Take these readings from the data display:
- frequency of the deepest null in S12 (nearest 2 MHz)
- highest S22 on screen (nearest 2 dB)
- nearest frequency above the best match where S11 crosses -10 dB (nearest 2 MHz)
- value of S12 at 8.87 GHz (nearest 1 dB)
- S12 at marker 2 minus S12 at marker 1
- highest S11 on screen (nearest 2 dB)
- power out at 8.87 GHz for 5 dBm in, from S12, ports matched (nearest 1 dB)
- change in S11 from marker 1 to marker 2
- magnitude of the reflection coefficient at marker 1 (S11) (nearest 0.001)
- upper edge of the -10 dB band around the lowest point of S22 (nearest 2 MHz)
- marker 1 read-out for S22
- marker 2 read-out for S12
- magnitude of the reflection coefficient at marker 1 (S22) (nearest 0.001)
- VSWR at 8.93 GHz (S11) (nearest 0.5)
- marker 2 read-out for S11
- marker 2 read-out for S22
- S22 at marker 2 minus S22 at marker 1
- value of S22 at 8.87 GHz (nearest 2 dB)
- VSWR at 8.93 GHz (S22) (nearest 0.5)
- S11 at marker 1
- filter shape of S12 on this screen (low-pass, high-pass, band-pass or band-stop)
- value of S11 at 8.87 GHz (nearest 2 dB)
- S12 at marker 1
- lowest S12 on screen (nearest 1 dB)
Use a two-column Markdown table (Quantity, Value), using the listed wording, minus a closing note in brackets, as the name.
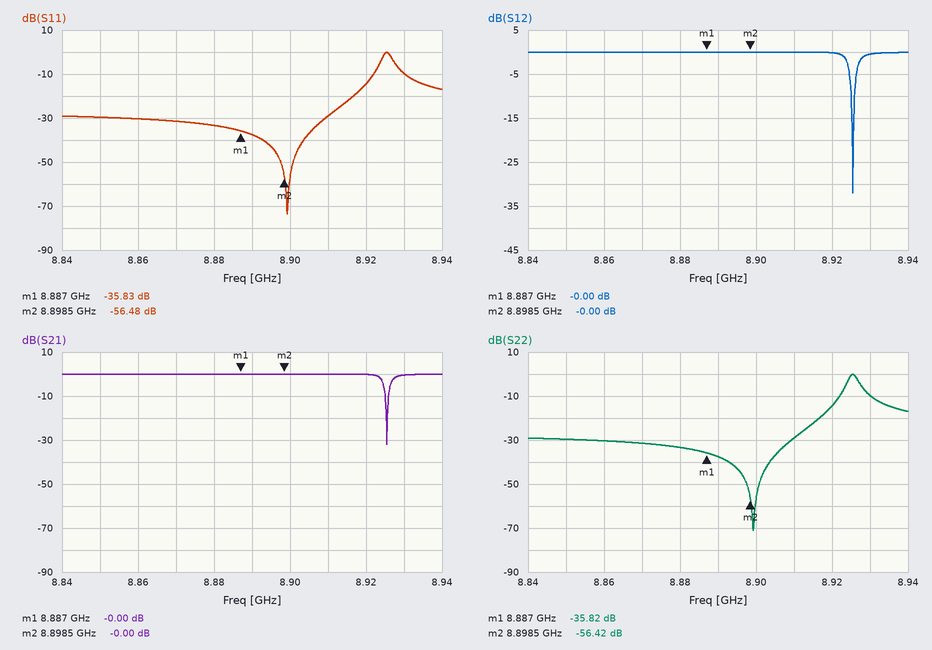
| Quantity | Value |
|---|---|
| frequency of the deepest null in S12 | 8.926 GHz |
| highest S22 on screen | 0 dB |
| nearest frequency above the best match where S11 crosses -10 dB | 8.922 GHz |
| value of S12 at 8.87 GHz | 0 dB |
| S12 at marker 2 minus S12 at marker 1 | 0.00 dB |
| highest S11 on screen | 0 dB |
| power out at 8.87 GHz for 5 dBm in, from S12, ports matched | 5 dBm |
| change in S11 from marker 1 to marker 2 | -20.65 dB |
| magnitude of the reflection coefficient at marker 1 (S11) | 0.016 |
| upper edge of the -10 dB band around the lowest point of S22 | 8.922 GHz |
| marker 1 read-out for S22 | -35.82 dB |
| marker 2 read-out for S12 | -0.00 dB |
| magnitude of the reflection coefficient at marker 1 (S22) | 0.016 |
| VSWR at 8.93 GHz (S11) | 2.0 |
| marker 2 read-out for S11 | -56.48 dB |
| marker 2 read-out for S22 | -56.42 dB |
| S22 at marker 2 minus S22 at marker 1 | -20.60 dB |
| value of S22 at 8.87 GHz | -32 dB |
| VSWR at 8.93 GHz (S22) | 2.0 |
| S11 at marker 1 | -35.83 dB |
| filter shape of S12 on this screen | band-stop |
| value of S11 at 8.87 GHz | -32 dB |
| S12 at marker 1 | -0.00 dB |
| lowest S12 on screen | -32 dB |
